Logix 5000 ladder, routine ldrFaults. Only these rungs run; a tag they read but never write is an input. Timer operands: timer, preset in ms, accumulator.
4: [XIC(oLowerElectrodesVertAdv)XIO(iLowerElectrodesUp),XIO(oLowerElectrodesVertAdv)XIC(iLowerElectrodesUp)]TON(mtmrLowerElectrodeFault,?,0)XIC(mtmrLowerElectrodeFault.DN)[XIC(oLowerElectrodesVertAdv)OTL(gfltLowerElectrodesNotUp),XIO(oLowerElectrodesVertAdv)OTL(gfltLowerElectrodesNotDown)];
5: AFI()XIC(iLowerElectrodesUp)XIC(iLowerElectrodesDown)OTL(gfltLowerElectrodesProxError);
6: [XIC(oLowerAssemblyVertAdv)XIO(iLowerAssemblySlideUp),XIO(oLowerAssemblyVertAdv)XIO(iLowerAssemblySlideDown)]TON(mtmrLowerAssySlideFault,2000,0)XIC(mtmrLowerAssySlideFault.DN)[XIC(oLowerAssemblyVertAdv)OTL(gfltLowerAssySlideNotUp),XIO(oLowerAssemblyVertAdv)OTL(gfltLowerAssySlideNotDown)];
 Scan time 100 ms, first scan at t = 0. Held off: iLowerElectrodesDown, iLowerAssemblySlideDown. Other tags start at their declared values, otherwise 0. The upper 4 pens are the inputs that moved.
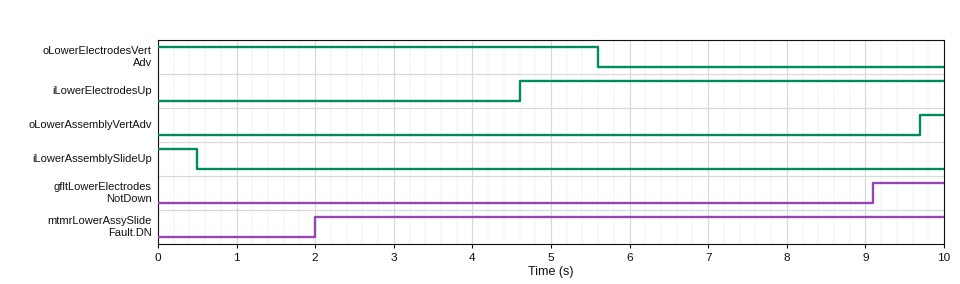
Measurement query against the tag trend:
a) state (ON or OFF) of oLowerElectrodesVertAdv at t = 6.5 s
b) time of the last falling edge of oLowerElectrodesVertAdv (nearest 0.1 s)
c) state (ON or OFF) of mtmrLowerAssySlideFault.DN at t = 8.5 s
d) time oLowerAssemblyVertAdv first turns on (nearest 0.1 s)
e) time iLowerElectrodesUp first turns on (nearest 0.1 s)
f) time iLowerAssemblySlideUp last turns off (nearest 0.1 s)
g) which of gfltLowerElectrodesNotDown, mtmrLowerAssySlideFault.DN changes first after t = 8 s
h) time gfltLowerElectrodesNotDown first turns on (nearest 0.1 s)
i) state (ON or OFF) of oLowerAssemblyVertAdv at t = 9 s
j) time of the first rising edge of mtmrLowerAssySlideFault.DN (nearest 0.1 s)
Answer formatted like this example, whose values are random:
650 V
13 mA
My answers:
OFF
5.6 s
ON
9.7 s
4.6 s
0.5 s
gfltLowerElectrodesNotDown
9.1 s
OFF
2.0 s
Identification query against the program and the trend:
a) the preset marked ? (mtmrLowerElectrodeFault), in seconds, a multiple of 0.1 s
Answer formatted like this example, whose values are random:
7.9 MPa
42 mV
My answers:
3.5 s
